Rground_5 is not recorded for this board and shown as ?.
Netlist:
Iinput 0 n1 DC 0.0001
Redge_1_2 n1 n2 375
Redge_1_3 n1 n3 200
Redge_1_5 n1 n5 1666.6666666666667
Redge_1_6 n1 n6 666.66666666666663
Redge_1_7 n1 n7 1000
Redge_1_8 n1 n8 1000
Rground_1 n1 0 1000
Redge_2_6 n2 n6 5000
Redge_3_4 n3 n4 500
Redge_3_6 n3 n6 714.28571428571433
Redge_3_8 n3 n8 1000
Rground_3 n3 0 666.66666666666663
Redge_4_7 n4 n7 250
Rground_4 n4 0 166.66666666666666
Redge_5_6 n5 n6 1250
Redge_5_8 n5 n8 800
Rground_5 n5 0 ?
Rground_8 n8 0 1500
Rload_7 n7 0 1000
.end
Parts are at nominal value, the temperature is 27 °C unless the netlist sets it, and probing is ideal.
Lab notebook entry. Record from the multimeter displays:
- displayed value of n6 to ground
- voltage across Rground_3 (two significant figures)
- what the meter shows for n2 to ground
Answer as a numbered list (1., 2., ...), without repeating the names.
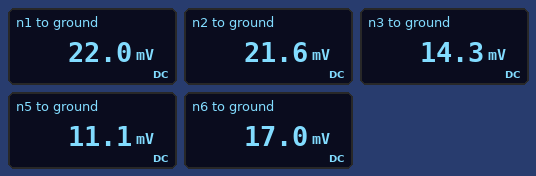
1. 17.0 mV
2. 14 mV
3. 21.6 mV
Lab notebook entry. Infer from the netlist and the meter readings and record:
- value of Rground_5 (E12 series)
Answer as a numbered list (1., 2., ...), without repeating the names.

1. 820 Ω
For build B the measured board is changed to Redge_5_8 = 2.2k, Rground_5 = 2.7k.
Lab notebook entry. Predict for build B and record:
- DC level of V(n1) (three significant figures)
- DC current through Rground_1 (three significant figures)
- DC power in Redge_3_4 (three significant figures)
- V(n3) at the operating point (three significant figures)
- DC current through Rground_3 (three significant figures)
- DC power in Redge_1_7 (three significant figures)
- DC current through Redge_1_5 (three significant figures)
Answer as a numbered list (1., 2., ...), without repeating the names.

1. 23.5 mV
2. 23.5 µA
3. 221 nW
4. 15.5 mV
5. 23.3 µA
6. 264 nW
7. 4.35 µA
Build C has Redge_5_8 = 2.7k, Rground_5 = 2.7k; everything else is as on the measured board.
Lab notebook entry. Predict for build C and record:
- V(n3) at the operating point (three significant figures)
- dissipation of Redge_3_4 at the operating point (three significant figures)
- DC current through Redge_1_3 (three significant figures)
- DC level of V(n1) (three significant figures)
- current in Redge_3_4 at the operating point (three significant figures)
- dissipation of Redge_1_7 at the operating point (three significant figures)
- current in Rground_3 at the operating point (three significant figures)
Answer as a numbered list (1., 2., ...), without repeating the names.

1. 15.5 mV
2. 221 nW
3. 39.9 µA
4. 23.5 mV
5. 21.0 µA
6. 264 nW
7. 23.3 µA
